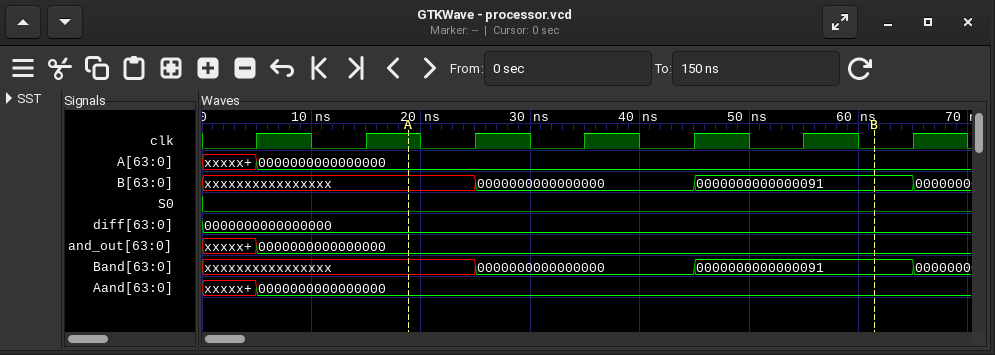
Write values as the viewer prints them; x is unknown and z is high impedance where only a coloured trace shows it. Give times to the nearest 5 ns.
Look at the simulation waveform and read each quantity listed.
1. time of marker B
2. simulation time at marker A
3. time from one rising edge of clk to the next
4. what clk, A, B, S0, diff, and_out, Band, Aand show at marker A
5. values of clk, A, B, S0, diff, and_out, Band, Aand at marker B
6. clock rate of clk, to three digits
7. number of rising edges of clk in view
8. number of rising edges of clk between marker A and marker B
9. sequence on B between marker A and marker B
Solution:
60 ns
20 ns
10 ns
clk=1, A=0000000000000000, B=xxxxxxxxxxxxxxxx, S0=0, diff=0000000000000000, and_out=0000000000000000, Band=xxxxxxxxxxxxxxxx, Aand=0000000000000000
clk=0, A=0000000000000000, B=0000000000000091, S0=0, diff=0000000000000000, and_out=0000000000000000, Band=0000000000000091, Aand=0000000000000000
100 MHz
7
4
xxxxxxxxxxxxxxxx, 0000000000000000, 0000000000000091
